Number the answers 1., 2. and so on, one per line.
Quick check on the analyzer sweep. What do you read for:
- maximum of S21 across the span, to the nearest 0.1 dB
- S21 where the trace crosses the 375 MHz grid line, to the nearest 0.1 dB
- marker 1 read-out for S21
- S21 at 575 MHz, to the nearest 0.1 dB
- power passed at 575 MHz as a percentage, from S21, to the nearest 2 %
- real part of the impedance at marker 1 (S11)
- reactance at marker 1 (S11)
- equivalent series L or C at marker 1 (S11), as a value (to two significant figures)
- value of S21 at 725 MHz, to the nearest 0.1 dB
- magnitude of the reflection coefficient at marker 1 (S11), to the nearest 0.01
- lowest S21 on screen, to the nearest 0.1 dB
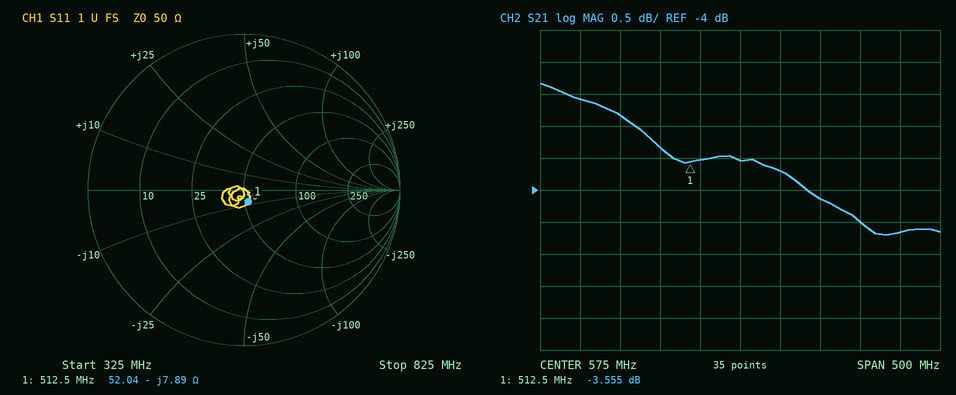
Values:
1. -2.3 dB
2. -2.6 dB
3. -3.555 dB
4. -3.5 dB
5. 44 %
6. 52.04 Ω
7. -7.89 Ω
8. 39 pF
9. -4.5 dB
10. 0.08
11. -4.7 dB
